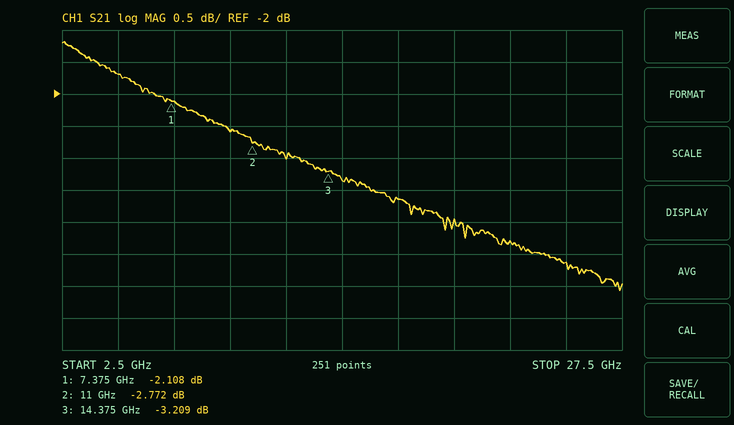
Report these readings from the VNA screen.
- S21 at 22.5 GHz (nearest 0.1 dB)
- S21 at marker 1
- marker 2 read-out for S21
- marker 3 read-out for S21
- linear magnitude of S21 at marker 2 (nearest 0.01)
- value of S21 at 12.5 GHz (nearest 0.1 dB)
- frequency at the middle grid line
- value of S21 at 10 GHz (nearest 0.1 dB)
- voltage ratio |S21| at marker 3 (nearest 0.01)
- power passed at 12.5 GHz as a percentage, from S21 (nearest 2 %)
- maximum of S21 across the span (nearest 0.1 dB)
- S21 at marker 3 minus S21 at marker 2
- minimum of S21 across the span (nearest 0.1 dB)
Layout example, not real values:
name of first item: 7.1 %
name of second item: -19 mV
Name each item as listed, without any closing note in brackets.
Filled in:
S21 at 22.5 GHz: -4.3 dB
S21 at marker 1: -2.108 dB
marker 2 read-out for S21: -2.772 dB
marker 3 read-out for S21: -3.209 dB
linear magnitude of S21 at marker 2: 0.73
value of S21 at 12.5 GHz: -3.0 dB
frequency at the middle grid line: 15 GHz
value of S21 at 10 GHz: -2.6 dB
voltage ratio |S21| at marker 3: 0.69
power passed at 12.5 GHz as a percentage, from S21: 50 %
maximum of S21 across the span: -1.2 dB
S21 at marker 3 minus S21 at marker 2: -0.437 dB
minimum of S21 across the span: -5.1 dB
